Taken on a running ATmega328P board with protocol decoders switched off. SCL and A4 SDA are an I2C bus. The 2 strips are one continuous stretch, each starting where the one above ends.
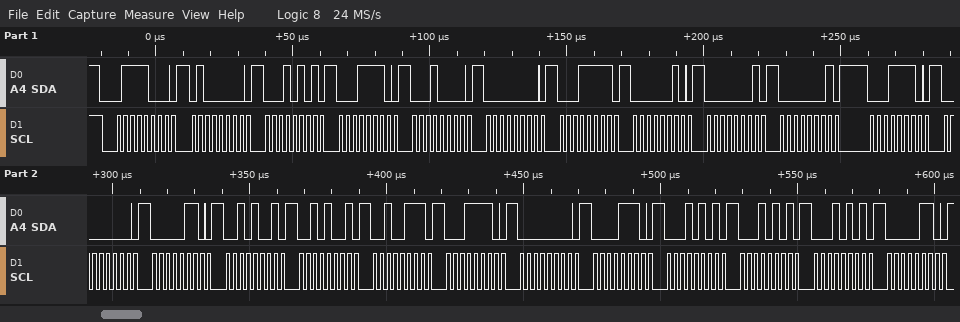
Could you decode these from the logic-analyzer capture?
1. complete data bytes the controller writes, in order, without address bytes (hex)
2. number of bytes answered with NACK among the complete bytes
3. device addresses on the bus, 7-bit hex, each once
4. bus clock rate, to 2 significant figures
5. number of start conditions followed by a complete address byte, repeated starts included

40 15 1E 10 00 1F 02 01 01 1E 00 06 29 29 27 1E 00 0E 15 15 15 06
0
0x3C
400 kHz
1
